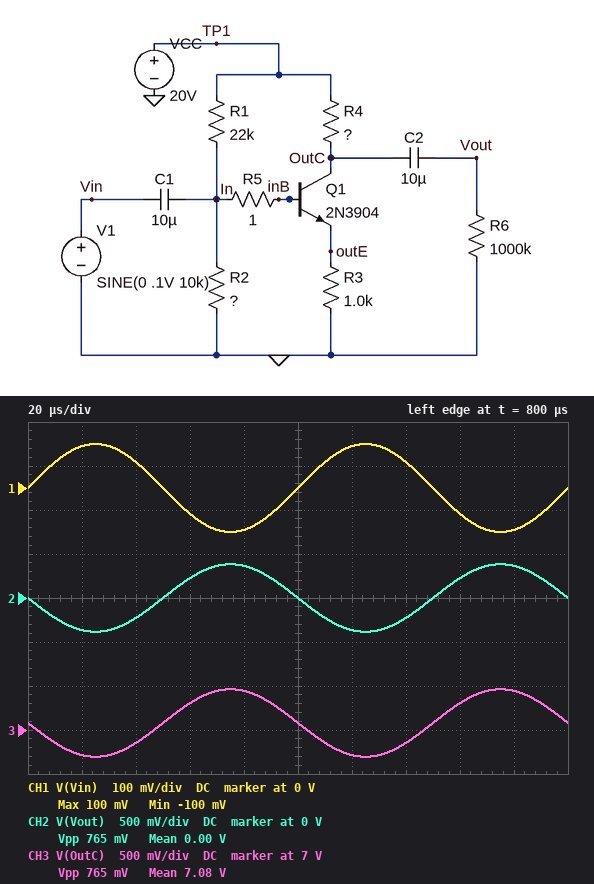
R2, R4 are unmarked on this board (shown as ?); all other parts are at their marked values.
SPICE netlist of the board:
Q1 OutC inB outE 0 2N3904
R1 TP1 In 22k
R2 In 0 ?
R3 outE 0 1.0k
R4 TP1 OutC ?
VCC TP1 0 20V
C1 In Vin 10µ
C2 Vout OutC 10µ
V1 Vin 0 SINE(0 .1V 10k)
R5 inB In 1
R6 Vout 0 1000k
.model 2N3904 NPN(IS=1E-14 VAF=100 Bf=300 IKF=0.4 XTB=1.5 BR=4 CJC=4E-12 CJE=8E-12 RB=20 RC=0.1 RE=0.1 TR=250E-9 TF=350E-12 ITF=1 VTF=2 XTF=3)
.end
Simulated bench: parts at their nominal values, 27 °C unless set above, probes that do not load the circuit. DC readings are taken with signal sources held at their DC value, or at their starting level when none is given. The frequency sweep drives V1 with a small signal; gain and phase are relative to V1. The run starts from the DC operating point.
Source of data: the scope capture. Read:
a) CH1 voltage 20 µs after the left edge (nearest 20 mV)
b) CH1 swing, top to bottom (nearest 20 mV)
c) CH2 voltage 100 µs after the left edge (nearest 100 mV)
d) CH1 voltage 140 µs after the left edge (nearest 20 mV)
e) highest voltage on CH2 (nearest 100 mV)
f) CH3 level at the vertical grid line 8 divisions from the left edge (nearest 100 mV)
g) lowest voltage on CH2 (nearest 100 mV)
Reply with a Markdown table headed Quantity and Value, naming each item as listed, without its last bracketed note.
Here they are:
| Quantity | Value |
|---|---|
| CH1 voltage 20 µs after the left edge | 100 mV |
| CH1 swing, top to bottom | 200 mV |
| CH2 voltage 100 µs after the left edge | 0 V |
| CH1 voltage 140 µs after the left edge | 60 mV |
| highest voltage on CH2 | 400 mV |
| CH3 level at the vertical grid line 8 divisions from the left edge | 7.3 V |
| lowest voltage on CH2 | -400 mV |
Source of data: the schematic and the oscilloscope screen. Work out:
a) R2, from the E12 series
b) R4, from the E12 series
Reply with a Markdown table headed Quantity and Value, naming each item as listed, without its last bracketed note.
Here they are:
| Quantity | Value |
|---|---|
| R2, from the E12 series | 5.6 kΩ |
| R4, from the E12 series | 3.9 kΩ |
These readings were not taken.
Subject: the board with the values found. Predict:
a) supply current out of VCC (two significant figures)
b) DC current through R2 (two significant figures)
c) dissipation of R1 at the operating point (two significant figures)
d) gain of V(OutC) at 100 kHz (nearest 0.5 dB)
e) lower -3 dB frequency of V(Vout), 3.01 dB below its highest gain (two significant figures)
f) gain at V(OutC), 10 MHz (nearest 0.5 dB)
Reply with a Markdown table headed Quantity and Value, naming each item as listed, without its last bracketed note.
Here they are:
| Quantity | Value |
|---|---|
| supply current out of VCC | 4.0 mA |
| DC current through R2 | 720 µA |
| dissipation of R1 at the operating point | 12 mW |
| gain of V(OutC) at 100 kHz | 11.5 dB |
| lower -3 dB frequency of V(Vout), 3.01 dB below its highest gain | 3.6 Hz |
| gain at V(OutC), 10 MHz | 10.5 dB |
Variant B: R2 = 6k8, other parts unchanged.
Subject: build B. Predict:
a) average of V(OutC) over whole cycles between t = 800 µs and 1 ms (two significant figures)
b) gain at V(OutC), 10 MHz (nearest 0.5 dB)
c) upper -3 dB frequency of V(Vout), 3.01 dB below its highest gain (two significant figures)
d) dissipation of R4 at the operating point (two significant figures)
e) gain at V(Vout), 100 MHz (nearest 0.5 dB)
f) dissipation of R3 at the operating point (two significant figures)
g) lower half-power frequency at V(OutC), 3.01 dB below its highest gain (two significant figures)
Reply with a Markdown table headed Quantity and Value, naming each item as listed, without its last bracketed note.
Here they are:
| Quantity | Value |
|---|---|
| average of V(OutC) over whole cycles between t = 800 µs and 1 ms | 4.6 V |
| gain at V(OutC), 10 MHz | 9.0 dB |
| upper -3 dB frequency of V(Vout), 3.01 dB below its highest gain | 11 MHz |
| dissipation of R4 at the operating point | 61 mW |
| gain at V(Vout), 100 MHz | 1.0 dB |
| dissipation of R3 at the operating point | 16 mW |
| lower half-power frequency at V(OutC), 3.01 dB below its highest gain | 3.1 Hz |
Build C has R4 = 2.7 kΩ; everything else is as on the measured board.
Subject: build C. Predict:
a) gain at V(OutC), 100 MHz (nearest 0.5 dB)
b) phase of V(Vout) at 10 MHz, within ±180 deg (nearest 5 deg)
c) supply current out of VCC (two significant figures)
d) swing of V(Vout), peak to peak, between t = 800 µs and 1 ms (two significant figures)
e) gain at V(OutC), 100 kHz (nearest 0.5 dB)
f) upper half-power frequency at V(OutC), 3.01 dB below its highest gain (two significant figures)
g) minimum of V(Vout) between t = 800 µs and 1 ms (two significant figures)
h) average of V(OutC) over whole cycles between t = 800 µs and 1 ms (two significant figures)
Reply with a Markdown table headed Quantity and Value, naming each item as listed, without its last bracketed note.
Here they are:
| Quantity | Value |
|---|---|
| gain at V(OutC), 100 MHz | 2.5 dB |
| phase of V(Vout) at 10 MHz, within ±180 deg | 155 deg |
| supply current out of VCC | 4.0 mA |
| swing of V(Vout), peak to peak, between t = 800 µs and 1 ms | 530 mV |
| gain at V(OutC), 100 kHz | 8.5 dB |
| upper half-power frequency at V(OutC), 3.01 dB below its highest gain | 39 MHz |
| minimum of V(Vout) between t = 800 µs and 1 ms | -270 mV |
| average of V(OutC) over whole cycles between t = 800 µs and 1 ms | 11 V |
